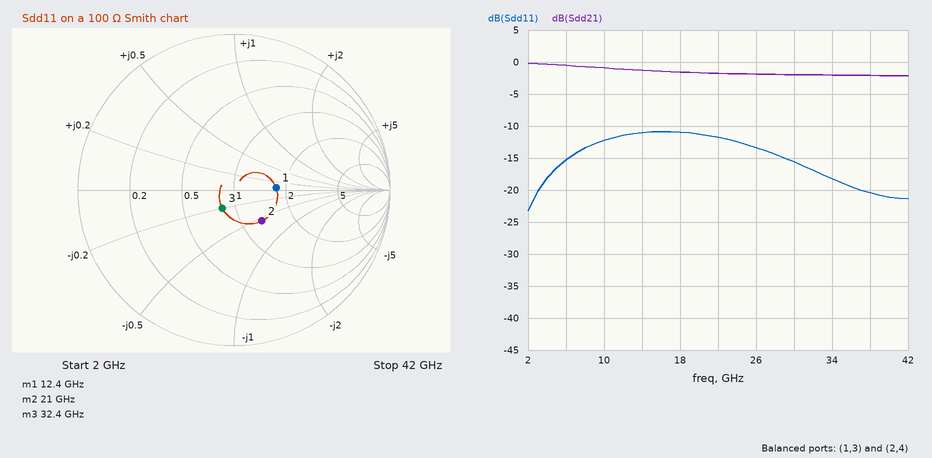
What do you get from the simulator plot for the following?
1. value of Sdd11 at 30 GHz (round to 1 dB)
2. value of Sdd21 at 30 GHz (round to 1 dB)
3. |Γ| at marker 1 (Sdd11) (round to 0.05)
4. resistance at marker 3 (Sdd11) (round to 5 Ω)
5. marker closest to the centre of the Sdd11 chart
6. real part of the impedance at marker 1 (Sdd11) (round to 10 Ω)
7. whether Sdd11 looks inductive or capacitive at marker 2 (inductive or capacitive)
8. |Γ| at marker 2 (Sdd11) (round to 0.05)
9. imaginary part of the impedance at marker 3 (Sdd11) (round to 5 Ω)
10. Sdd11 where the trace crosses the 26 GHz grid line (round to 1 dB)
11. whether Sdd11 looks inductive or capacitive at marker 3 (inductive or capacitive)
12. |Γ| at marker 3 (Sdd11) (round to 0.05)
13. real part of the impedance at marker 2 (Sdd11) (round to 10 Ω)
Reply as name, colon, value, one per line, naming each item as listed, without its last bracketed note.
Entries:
value of Sdd11 at 30 GHz: -16 dB
value of Sdd21 at 30 GHz: -2 dB
|Γ| at marker 1 (Sdd11): 0.25
resistance at marker 3 (Sdd11): 85 Ω
marker closest to the centre of the Sdd11 chart: marker 3
real part of the impedance at marker 1 (Sdd11): 170 Ω
whether Sdd11 looks inductive or capacitive at marker 2: capacitive
|Γ| at marker 2 (Sdd11): 0.25
imaginary part of the impedance at marker 3 (Sdd11): -20 Ω
Sdd11 where the trace crosses the 26 GHz grid line: -13 dB
whether Sdd11 looks inductive or capacitive at marker 3: capacitive
|Γ| at marker 3 (Sdd11): 0.15
real part of the impedance at marker 2 (Sdd11): 130 Ω
